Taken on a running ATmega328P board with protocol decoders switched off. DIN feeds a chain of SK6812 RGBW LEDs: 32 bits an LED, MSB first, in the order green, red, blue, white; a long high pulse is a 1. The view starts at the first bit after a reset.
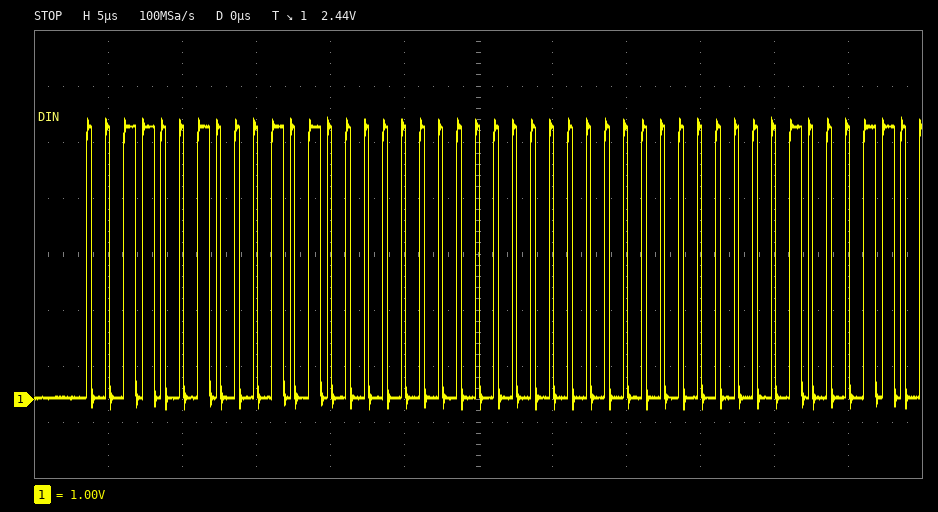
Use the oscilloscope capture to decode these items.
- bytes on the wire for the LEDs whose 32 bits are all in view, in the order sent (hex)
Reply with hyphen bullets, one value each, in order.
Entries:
- 32 28 00 00
